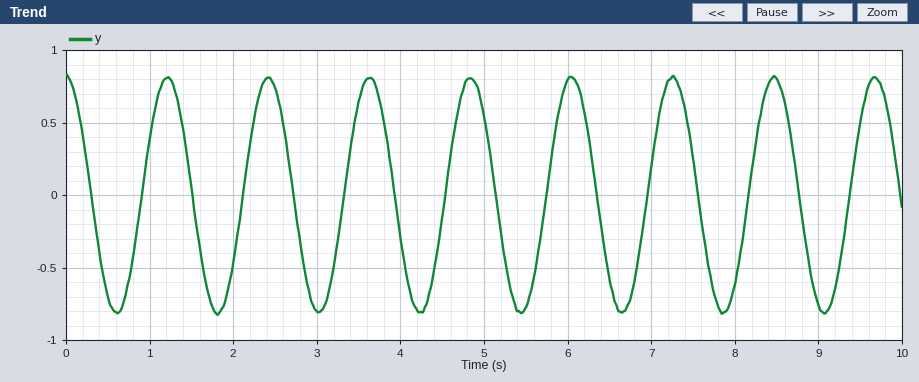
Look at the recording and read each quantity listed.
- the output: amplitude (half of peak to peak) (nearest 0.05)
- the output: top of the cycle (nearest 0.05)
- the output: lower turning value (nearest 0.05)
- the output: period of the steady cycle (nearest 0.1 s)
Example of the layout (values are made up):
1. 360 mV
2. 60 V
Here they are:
1. 0.80
2. 0.80
3. -0.80
4. 1.2 s
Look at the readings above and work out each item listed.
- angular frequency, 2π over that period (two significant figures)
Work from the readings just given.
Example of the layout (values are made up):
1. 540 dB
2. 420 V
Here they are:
1. 5.2 rad/s
